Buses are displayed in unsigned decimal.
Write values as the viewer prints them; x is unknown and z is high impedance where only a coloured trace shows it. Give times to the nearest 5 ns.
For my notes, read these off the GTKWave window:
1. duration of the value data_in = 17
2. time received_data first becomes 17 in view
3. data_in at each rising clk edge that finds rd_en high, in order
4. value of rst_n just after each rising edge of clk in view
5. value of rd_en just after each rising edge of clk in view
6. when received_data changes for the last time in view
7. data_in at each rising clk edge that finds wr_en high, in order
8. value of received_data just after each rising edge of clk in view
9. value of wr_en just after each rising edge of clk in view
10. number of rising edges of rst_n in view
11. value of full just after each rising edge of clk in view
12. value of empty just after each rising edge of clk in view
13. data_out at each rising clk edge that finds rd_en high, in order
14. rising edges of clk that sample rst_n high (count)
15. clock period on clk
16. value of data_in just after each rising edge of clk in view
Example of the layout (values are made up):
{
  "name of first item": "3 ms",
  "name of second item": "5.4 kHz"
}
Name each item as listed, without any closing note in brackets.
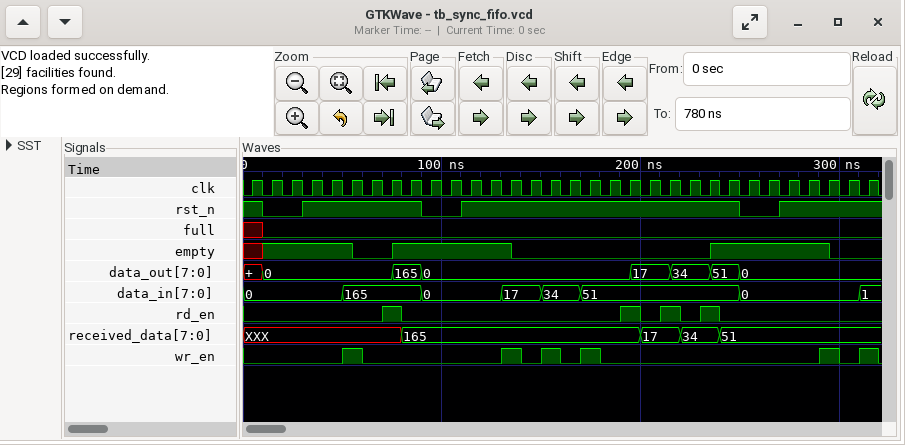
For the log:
{
  "duration of the value data_in = 17": "20 ns",
  "time received_data first becomes 17 in view": "200 ns",
  "data_in at each rising clk edge that finds rd_en high, in order": "165, 51, 51, 51",
  "value of rst_n just after each rising edge of clk in view": "1 0 0 1 1 1 1 1 1 0 0 1 1 1 1 1 1 1 1 1 1 1 1 1 1 0 0 1 1 1 1 1",
  "value of rd_en just after each rising edge of clk in view": "0 0 0 0 0 0 0 1 0 0 0 0 0 0 0 0 0 0 0 1 0 1 0 1 0 0 0 0 0 0 0 0",
  "when received_data changes for the last time in view": "240 ns",
  "data_in at each rising clk edge that finds wr_en high, in order": "165, 17, 34, 51, 0, 1",
  "value of received_data just after each rising edge of clk in view": "XXX, XXX, XXX, XXX, XXX, XXX, XXX, XXX, 165, 165, 165, 165, 165, 165, 165, 165, 165, 165, 165, 165, 17, 17, 34, 34, 51, 51, 51, 51, 51, 51, 51, 51",
  "value of wr_en just after each rising edge of clk in view": "0 0 0 0 0 1 0 0 0 0 0 0 0 1 0 1 0 1 0 0 0 0 0 0 0 0 0 0 0 1 0 1",
  "number of rising edges of rst_n in view": "3",
  "value of full just after each rising edge of clk in view": "x 0 0 0 0 0 0 0 0 0 0 0 0 0 0 0 0 0 0 0 0 0 0 0 0 0 0 0 0 0 0 0",
  "value of empty just after each rising edge of clk in view": "x 1 1 1 1 0 0 1 1 1 1 1 1 0 0 0 0 0 0 0 0 0 0 1 1 1 1 1 1 0 0 0",
  "data_out at each rising clk edge that finds rd_en high, in order": "0, 0, 17, 34",
  "rising edges of clk that sample rst_n high": "26",
  "clock period on clk": "10 ns",
  "value of data_in just after each rising edge of clk in view": "0, 0, 0, 0, 0, 165, 165, 165, 165, 0, 0, 0, 0, 17, 17, 34, 34, 51, 51, 51, 51, 51, 51, 51, 51, 0, 0, 0, 0, 0, 0, 1"
}
